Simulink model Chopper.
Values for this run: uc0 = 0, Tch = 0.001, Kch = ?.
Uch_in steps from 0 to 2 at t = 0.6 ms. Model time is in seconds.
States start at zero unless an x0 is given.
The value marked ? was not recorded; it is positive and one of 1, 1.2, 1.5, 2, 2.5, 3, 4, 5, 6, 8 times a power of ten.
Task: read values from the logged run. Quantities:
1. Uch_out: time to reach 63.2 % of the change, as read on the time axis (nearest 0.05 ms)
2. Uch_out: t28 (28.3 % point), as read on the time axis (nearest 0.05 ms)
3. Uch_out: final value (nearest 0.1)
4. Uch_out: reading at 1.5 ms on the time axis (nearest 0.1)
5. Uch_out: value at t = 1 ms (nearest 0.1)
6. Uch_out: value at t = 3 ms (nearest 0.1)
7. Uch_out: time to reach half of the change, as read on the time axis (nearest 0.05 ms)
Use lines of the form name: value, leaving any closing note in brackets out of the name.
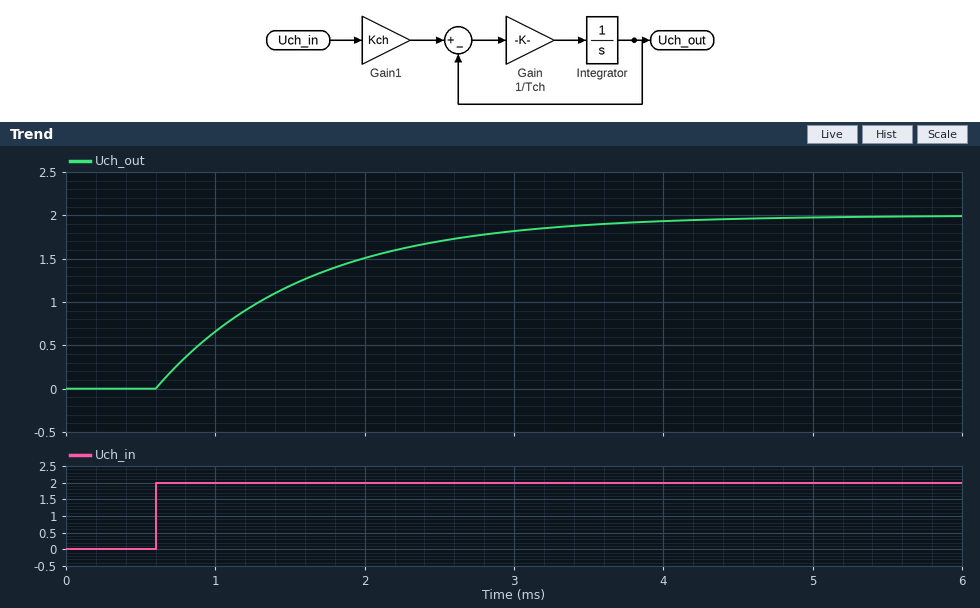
Uch_out: time to reach 63.2 % of the change, as read on the time axis: 1.60 ms
Uch_out: t28 (28.3 % point), as read on the time axis: 0.95 ms
Uch_out: final value: 2.0
Uch_out: reading at 1.5 ms on the time axis: 1.2
Uch_out: value at t = 1 ms: 0.7
Uch_out: value at t = 3 ms: 1.8
Uch_out: time to reach half of the change, as read on the time axis: 1.30 ms
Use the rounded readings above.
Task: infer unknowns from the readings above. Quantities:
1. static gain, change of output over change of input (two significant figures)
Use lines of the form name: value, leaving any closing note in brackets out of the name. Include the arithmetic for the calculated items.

static gain, change of output over change of input: (2 - 0) / (2 - 0) = 1.0
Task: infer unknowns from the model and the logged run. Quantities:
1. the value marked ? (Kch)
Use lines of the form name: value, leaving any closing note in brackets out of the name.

the value marked ?: 1
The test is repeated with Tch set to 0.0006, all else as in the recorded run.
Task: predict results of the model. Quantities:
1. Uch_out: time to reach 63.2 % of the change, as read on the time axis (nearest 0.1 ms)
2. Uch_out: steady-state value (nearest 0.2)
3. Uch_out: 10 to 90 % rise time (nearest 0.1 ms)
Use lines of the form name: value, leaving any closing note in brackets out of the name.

Uch_out: time to reach 63.2 % of the change, as read on the time axis: 1.2 ms
Uch_out: steady-state value: 2.0
Uch_out: 10 to 90 % rise time: 1.3 ms
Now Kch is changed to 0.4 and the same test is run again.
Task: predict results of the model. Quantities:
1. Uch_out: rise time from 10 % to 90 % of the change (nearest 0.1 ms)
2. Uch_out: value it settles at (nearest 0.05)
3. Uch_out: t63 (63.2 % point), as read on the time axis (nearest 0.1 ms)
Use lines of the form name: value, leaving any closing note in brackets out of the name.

Uch_out: rise time from 10 % to 90 % of the change: 2.2 ms
Uch_out: value it settles at: 0.80
Uch_out: t63 (63.2 % point), as read on the time axis: 1.6 ms
